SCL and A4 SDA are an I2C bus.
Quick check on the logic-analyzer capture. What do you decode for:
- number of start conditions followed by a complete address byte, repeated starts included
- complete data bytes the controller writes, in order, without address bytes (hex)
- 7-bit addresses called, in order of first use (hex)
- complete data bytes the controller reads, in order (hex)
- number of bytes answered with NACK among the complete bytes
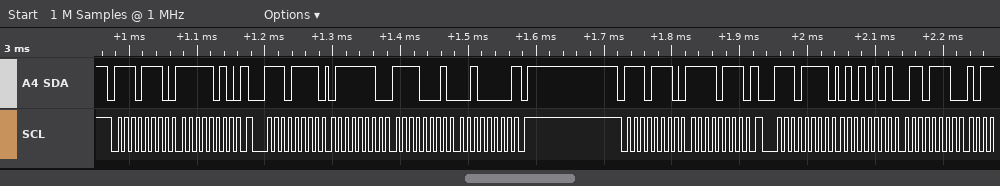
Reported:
4
FA F7
0x77
7E F1 20 55 6E
1
